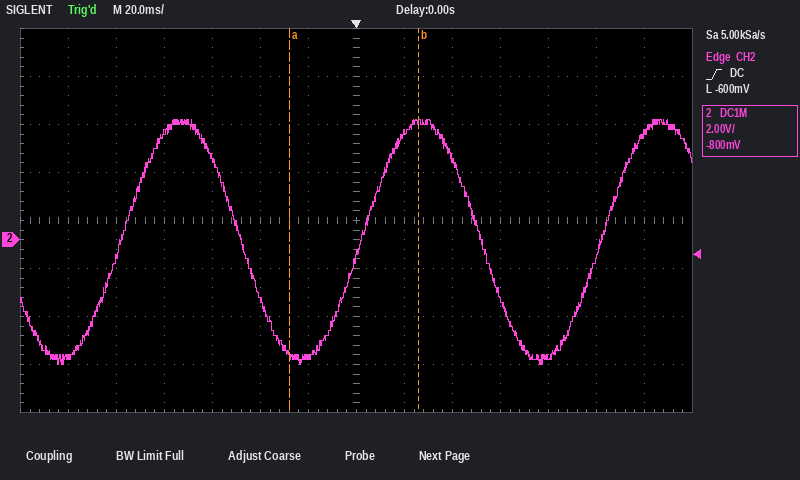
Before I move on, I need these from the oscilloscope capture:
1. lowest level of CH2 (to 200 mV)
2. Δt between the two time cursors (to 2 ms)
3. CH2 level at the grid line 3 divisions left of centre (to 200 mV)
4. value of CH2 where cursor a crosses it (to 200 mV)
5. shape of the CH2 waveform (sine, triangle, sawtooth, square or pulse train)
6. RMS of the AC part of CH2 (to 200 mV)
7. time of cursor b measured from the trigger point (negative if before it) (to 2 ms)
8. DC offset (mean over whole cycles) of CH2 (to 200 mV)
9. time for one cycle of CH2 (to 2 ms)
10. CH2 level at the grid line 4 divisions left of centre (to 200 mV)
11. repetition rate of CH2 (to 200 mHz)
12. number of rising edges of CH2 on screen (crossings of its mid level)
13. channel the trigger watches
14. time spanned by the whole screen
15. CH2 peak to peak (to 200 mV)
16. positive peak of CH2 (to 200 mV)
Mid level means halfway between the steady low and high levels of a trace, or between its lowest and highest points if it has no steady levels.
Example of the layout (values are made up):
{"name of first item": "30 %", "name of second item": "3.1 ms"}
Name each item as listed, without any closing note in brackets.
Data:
{"lowest level of CH2": "-5.2 V", "Δt between the two time cursors": "54 ms", "CH2 level at the grid line 3 divisions left of centre": "3.4 V", "value of CH2 where cursor a crosses it": "-4.8 V", "shape of the CH2 waveform": "sine", "RMS of the AC part of CH2": "3.6 V", "time of cursor b measured from the trigger point (negative if before it)": "+26 ms", "DC offset (mean over whole cycles) of CH2": "0.0 V", "time for one cycle of CH2": "100 ms", "CH2 level at the grid line 4 divisions left of centre": "4.4 V", "repetition rate of CH2": "10.0 Hz", "number of rising edges of CH2 on screen": "3", "channel the trigger watches": "CH2", "time spanned by the whole screen": "280 ms", "CH2 peak to peak": "10.2 V", "positive peak of CH2": "5.0 V"}
